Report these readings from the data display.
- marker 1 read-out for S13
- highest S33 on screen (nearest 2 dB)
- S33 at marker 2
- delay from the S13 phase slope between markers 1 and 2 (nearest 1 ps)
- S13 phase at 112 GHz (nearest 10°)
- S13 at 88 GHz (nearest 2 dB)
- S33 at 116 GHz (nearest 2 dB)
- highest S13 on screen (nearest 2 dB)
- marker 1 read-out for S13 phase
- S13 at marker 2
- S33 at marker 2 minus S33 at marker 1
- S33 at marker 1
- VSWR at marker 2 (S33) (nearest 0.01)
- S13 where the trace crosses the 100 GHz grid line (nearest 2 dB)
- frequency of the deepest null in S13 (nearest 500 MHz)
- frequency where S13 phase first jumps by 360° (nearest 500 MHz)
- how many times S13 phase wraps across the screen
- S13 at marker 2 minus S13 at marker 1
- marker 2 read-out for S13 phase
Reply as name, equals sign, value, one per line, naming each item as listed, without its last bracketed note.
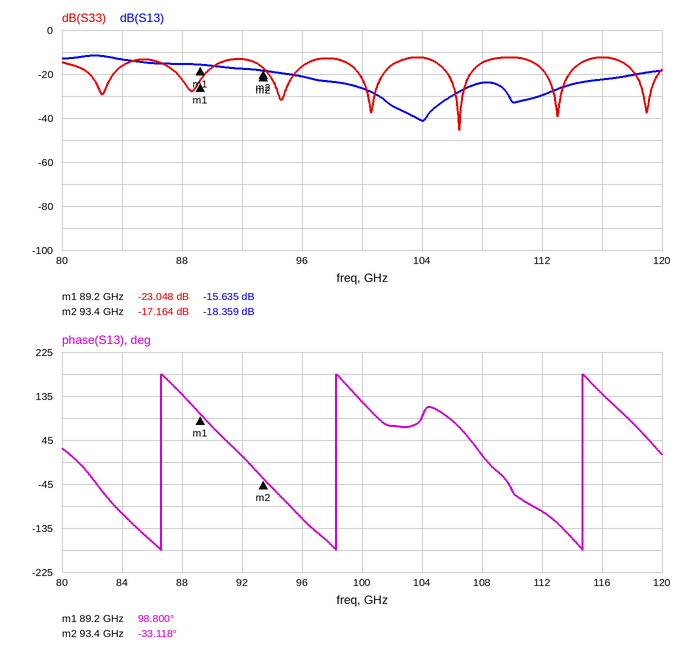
marker 1 read-out for S13 = -15.635 dB
highest S33 on screen = -12 dB
S33 at marker 2 = -17.164 dB
delay from the S13 phase slope between markers 1 and 2 = 87 ps
S13 phase at 112 GHz = -100°
S13 at 88 GHz = -16 dB
S33 at 116 GHz = -12 dB
highest S13 on screen = -12 dB
marker 1 read-out for S13 phase = 98.800°
S13 at marker 2 = -18.359 dB
S33 at marker 2 minus S33 at marker 1 = 5.884 dB
S33 at marker 1 = -23.048 dB
VSWR at marker 2 (S33) = 1.32
S13 where the trace crosses the 100 GHz grid line = -26 dB
frequency of the deepest null in S13 = 104.0 GHz
frequency where S13 phase first jumps by 360° = 86.5 GHz
how many times S13 phase wraps across the screen = 3
S13 at marker 2 minus S13 at marker 1 = -2.724 dB
marker 2 read-out for S13 phase = -33.118°
